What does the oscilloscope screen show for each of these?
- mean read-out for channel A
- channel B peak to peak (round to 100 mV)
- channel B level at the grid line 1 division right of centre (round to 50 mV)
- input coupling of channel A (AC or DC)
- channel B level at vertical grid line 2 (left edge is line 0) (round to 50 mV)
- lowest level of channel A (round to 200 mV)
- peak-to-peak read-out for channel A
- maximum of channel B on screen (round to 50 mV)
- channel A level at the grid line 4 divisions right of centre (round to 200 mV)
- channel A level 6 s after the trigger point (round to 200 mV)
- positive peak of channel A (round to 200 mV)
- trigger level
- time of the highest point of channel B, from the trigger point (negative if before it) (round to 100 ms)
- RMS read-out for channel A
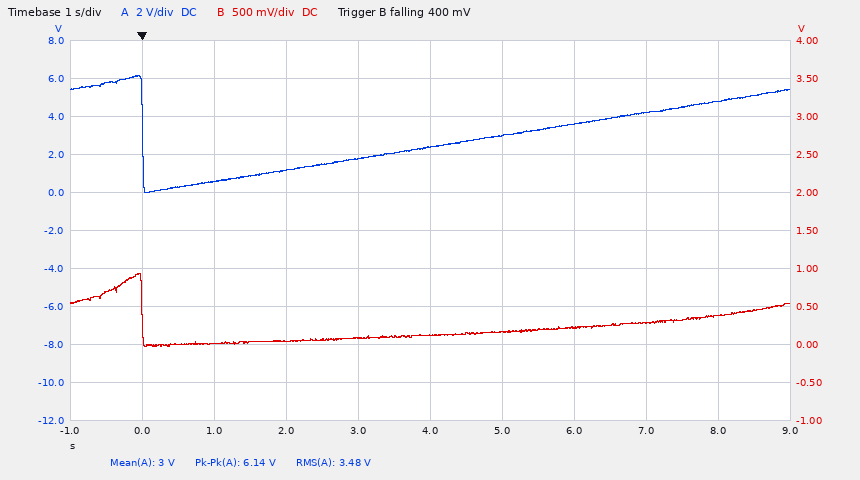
3 V
1.00 V
150 mV
DC
0 mV
0.0 V
6.14 V
950 mV
4.8 V
3.6 V
6.2 V
400 mV
-100 ms
3.48 V
